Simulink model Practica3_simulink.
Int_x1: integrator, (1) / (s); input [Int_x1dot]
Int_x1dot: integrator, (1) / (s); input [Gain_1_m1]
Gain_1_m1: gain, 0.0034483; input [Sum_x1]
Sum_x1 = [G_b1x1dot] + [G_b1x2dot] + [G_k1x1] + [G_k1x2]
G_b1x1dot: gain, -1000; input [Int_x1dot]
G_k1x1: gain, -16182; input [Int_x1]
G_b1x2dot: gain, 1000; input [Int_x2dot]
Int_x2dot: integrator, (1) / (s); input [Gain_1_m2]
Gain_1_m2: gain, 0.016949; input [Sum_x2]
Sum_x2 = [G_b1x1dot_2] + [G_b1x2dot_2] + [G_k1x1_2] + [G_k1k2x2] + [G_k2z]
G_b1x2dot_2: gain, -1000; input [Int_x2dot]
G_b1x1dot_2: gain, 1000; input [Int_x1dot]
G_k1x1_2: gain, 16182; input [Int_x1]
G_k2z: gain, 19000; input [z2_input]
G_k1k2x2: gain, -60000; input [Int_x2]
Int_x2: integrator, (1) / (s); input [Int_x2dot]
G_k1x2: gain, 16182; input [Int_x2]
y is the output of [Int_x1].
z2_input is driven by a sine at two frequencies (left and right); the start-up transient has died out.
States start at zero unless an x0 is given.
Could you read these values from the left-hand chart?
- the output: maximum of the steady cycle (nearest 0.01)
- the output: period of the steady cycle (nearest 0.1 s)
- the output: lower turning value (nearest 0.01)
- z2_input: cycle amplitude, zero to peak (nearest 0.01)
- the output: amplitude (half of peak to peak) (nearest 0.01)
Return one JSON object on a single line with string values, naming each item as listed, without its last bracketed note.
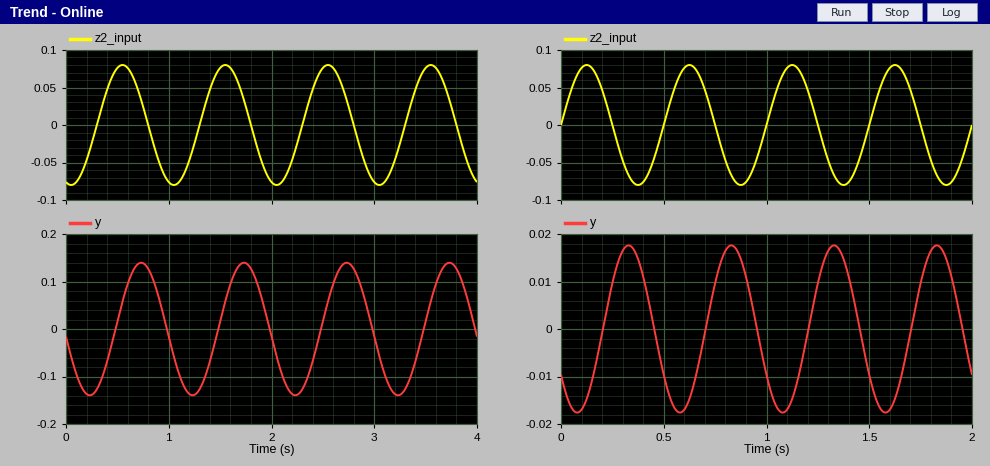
{"the output: maximum of the steady cycle": "0.14", "the output: period of the steady cycle": "1.0 s", "the output: lower turning value": "-0.14", "z2_input: cycle amplitude, zero to peak": "0.08", "the output: amplitude (half of peak to peak)": "0.14"}
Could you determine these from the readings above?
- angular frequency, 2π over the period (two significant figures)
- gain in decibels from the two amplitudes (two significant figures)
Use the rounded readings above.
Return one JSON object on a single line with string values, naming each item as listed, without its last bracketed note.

{"angular frequency, 2π over the period": "6.3 rad/s", "gain in decibels from the two amplitudes": "4.9 dB"}
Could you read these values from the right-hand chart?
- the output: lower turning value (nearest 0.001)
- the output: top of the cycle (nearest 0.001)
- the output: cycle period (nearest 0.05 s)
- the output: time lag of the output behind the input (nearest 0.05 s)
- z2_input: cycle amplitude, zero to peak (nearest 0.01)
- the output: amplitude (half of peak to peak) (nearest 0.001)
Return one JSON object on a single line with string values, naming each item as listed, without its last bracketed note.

{"the output: lower turning value": "-0.018", "the output: top of the cycle": "0.018", "the output: cycle period": "0.50 s", "the output: time lag of the output behind the input": "0.20 s", "z2_input: cycle amplitude, zero to peak": "0.08", "the output: amplitude (half of peak to peak)": "0.018"}
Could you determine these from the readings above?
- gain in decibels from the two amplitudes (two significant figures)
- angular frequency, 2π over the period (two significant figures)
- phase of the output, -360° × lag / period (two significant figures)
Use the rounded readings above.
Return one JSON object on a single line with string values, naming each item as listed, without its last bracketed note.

{"gain in decibels from the two amplitudes": "-13 dB", "angular frequency, 2π over the period": "13 rad/s", "phase of the output, -360° × lag / period": "-140°"}
